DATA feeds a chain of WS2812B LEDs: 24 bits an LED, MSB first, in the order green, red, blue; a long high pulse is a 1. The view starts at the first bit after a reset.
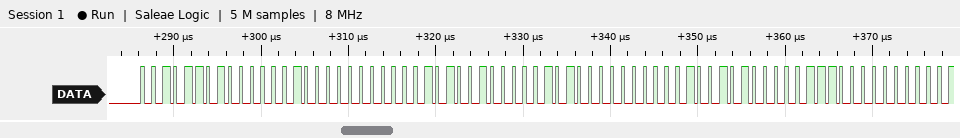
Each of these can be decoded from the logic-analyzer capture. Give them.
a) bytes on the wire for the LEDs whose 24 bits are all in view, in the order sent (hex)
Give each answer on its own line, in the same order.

2D 02 00 29 05 00 25 07 00
